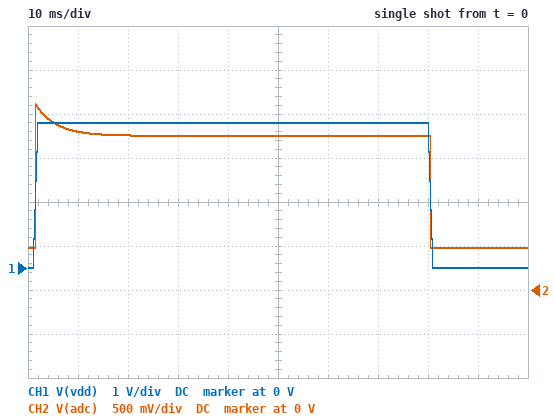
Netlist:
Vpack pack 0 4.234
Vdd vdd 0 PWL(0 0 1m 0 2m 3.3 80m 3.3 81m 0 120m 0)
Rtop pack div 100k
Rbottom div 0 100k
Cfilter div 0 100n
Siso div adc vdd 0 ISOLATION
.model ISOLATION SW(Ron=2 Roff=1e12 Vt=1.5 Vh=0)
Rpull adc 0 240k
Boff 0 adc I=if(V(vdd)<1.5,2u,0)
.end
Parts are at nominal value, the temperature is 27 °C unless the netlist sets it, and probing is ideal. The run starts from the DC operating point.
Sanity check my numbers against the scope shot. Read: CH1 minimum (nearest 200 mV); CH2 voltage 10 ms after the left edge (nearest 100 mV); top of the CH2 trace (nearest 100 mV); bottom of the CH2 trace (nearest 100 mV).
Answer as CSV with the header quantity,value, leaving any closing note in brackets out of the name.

quantity,value
CH1 minimum,0 V
CH2 voltage 10 ms after the left edge,1.8 V
top of the CH2 trace,2.1 V
bottom of the CH2 trace,500 mV
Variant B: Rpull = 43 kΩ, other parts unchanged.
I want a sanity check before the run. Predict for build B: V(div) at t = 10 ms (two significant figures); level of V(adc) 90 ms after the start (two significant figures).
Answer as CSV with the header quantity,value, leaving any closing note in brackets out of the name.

quantity,value
V(div) at t = 10 ms,1.0 V
level of V(adc) 90 ms after the start,86 mV
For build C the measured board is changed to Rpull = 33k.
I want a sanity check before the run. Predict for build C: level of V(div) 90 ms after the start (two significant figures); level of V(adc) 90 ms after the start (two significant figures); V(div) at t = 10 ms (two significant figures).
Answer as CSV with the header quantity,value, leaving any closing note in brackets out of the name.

quantity,value
level of V(div) 90 ms after the start,1.9 V
level of V(adc) 90 ms after the start,66 mV
V(div) at t = 10 ms,860 mV
